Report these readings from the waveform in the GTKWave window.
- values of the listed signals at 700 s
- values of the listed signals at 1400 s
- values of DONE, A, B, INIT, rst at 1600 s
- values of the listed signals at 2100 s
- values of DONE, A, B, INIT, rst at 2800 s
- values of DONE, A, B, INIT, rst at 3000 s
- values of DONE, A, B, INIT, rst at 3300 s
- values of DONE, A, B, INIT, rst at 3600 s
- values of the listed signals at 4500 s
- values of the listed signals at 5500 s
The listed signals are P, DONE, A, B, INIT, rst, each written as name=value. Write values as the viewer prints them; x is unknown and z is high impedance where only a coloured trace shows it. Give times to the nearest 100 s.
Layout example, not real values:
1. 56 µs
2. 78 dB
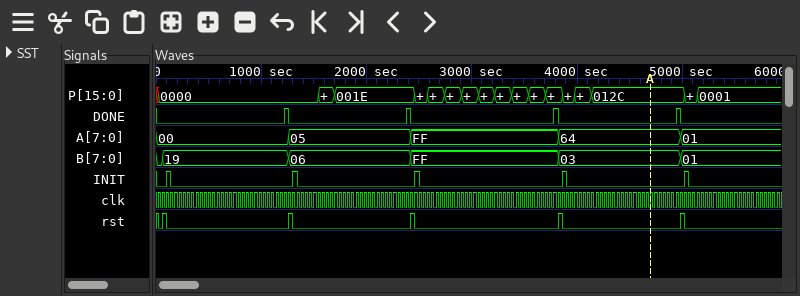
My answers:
1. P=0000, DONE=0, A=00, B=19, INIT=0, rst=0
2. P=0000, DONE=0, A=05, B=06, INIT=0, rst=0
3. DONE=0, A=05, B=06, INIT=0, rst=0
4. P=001E, DONE=0, A=05, B=06, INIT=0, rst=0
5. DONE=0, A=FF, B=FF, INIT=0, rst=0
6. DONE=0, A=FF, B=FF, INIT=0, rst=0
7. DONE=0, A=FF, B=FF, INIT=0, rst=0
8. DONE=0, A=FF, B=FF, INIT=0, rst=0
9. P=012C, DONE=0, A=64, B=03, INIT=0, rst=0
10. P=0001, DONE=0, A=01, B=01, INIT=0, rst=0
